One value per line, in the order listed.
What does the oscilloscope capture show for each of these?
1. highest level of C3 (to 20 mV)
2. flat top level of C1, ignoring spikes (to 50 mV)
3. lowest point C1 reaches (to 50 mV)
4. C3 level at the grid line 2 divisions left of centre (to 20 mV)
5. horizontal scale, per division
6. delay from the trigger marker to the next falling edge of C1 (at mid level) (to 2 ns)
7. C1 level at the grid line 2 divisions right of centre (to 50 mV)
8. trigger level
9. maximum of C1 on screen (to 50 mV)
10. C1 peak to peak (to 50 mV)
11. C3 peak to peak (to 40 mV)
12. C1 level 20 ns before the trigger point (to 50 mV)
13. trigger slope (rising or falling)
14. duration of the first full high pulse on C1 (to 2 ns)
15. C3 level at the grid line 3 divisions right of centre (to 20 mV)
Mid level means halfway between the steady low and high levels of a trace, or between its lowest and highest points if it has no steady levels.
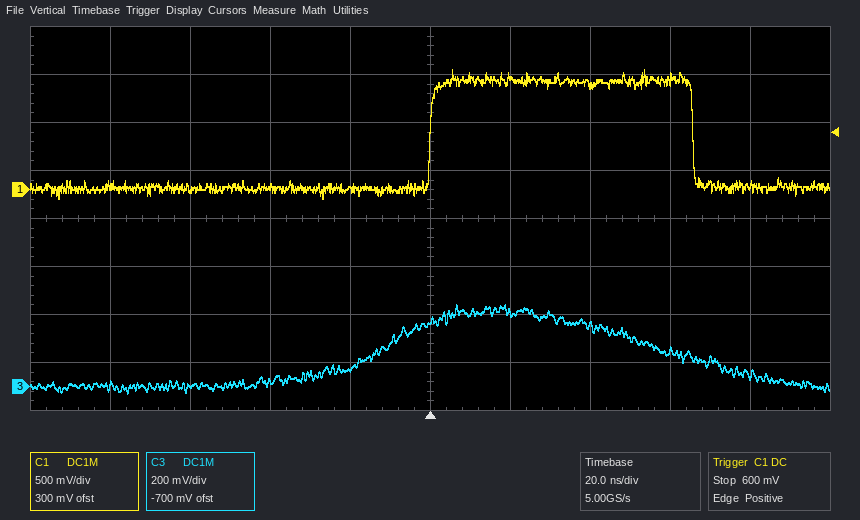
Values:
340 mV
1.15 V
-100 mV
20 mV
20 ns
66 ns
1.10 V
600 mV
1.25 V
1.35 V
360 mV
0 mV
rising
66 ns
140 mV
